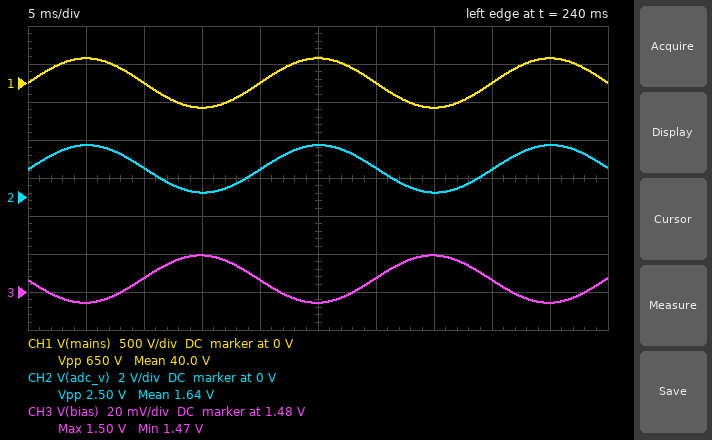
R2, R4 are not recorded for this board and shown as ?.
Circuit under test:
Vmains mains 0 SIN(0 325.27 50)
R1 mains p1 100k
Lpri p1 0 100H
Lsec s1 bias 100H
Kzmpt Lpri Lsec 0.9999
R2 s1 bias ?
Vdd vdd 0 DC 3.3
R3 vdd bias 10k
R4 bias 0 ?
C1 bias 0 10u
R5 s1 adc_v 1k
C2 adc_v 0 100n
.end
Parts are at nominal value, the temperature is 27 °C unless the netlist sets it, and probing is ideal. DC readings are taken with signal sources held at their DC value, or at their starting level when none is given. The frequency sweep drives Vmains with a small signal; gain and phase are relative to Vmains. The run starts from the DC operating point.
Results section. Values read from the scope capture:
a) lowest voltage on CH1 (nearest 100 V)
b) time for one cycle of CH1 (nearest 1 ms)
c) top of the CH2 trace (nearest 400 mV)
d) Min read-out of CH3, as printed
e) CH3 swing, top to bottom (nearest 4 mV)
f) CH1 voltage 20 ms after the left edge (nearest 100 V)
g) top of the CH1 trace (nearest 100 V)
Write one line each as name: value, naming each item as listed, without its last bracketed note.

lowest voltage on CH1: -300 V
time for one cycle of CH1: 20 ms
top of the CH2 trace: 2.8 V
Min read-out of CH3, as printed: 1.47 V
CH3 swing, top to bottom: 24 mV
CH1 voltage 20 ms after the left edge: 0 V
top of the CH1 trace: 300 V
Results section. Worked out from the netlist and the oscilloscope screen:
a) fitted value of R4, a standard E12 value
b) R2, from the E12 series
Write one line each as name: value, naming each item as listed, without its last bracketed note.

fitted value of R4, a standard E12 value: 8.2 kΩ
R2, from the E12 series: 390 Ω
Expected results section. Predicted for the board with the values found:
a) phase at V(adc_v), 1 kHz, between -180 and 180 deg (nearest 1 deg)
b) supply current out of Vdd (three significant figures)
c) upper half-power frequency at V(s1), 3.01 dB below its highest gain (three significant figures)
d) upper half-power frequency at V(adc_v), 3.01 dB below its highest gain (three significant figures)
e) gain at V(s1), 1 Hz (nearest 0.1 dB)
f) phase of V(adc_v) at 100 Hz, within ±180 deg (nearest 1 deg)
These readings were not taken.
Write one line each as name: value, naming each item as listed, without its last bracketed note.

phase at V(adc_v), 1 kHz, between -180 and 180 deg: -41 deg
supply current out of Vdd: 181 µA
upper half-power frequency at V(s1), 3.01 dB below its highest gain: 193 kHz
upper half-power frequency at V(adc_v), 3.01 dB below its highest gain: 1.16 kHz
gain at V(s1), 1 Hz: -49.6 dB
phase of V(adc_v) at 100 Hz, within ±180 deg: -5 deg
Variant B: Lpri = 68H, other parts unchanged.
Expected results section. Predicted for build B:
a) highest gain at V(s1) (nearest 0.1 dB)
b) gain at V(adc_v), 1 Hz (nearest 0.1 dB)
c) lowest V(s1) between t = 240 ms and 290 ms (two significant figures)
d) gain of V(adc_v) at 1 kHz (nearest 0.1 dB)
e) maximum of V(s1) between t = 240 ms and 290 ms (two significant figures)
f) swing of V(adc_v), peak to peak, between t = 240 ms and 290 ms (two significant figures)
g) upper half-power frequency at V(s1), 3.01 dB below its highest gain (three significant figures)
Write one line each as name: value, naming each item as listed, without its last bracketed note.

highest gain at V(s1): -50.0 dB
gain at V(adc_v), 1 Hz: -51.3 dB
lowest V(s1) between t = 240 ms and 290 ms: 450 mV
gain of V(adc_v) at 1 kHz: -52.4 dB
maximum of V(s1) between t = 240 ms and 290 ms: 2.5 V
swing of V(adc_v), peak to peak, between t = 240 ms and 290 ms: 2.1 V
upper half-power frequency at V(s1), 3.01 dB below its highest gain: 282 kHz
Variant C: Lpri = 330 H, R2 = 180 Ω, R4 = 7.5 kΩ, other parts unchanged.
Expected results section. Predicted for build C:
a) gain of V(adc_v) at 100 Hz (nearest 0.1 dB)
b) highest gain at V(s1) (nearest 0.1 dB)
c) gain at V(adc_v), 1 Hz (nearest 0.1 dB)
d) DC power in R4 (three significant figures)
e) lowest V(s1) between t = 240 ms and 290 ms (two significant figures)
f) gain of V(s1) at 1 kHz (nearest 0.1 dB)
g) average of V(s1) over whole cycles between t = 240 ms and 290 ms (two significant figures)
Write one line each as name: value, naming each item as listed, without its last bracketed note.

gain of V(adc_v) at 100 Hz: -49.9 dB
highest gain at V(s1): -49.8 dB
gain at V(adc_v), 1 Hz: -50.1 dB
DC power in R4: 267 µW
lowest V(s1) between t = 240 ms and 290 ms: 360 mV
gain of V(s1) at 1 kHz: -50.3 dB
average of V(s1) over whole cycles between t = 240 ms and 290 ms: 1.4 V
